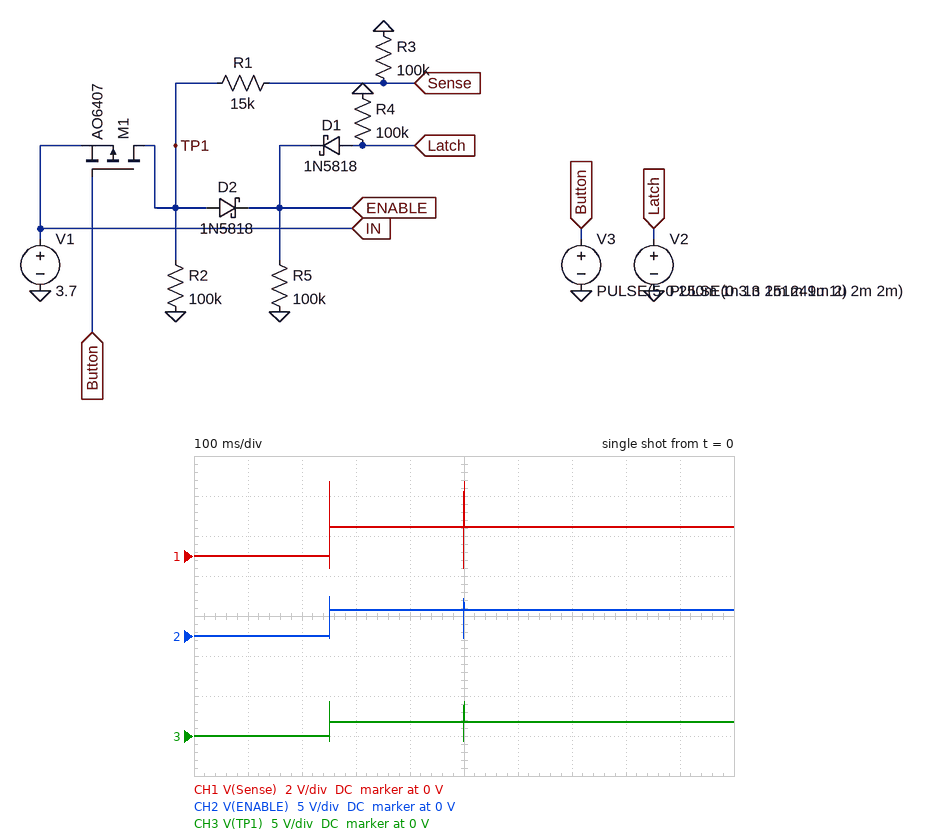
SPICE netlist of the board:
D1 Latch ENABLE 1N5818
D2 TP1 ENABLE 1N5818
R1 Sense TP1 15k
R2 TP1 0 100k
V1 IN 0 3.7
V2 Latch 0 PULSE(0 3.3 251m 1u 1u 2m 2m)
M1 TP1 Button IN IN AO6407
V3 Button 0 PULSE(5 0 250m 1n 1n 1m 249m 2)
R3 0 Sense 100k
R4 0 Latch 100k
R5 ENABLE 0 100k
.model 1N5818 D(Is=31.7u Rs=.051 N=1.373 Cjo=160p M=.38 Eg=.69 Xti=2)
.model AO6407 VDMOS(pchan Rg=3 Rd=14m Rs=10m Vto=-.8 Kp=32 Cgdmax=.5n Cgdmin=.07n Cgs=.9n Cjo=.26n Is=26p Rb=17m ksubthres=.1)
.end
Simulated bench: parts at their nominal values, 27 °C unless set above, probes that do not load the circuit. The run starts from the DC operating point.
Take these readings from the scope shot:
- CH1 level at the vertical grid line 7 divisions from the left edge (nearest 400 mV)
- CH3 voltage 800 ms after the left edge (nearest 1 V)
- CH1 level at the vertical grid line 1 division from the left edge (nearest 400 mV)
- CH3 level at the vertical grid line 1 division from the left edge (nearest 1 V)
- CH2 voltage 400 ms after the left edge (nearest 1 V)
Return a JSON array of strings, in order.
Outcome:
["1.6 V", "2 V", "0 V", "0 V", "3 V"]
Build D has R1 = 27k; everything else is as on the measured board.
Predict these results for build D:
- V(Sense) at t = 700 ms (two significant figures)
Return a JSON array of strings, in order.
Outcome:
["1.4 V"]
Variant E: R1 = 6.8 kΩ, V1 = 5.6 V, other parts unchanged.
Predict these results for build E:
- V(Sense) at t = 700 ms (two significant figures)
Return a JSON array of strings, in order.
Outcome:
["5.2 V"]
